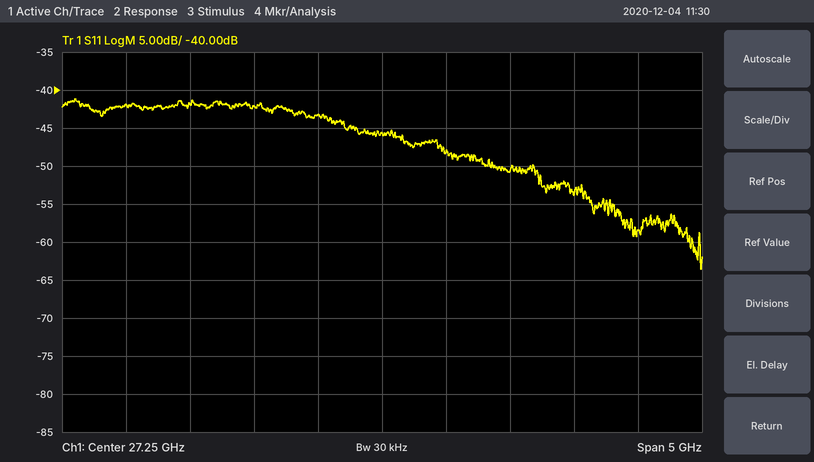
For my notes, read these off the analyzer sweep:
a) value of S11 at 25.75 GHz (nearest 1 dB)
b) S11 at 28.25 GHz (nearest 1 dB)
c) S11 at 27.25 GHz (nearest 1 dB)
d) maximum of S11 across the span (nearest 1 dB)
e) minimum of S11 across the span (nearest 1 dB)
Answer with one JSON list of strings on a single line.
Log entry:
["-42 dB", "-51 dB", "-46 dB", "-41 dB", "-64 dB"]
